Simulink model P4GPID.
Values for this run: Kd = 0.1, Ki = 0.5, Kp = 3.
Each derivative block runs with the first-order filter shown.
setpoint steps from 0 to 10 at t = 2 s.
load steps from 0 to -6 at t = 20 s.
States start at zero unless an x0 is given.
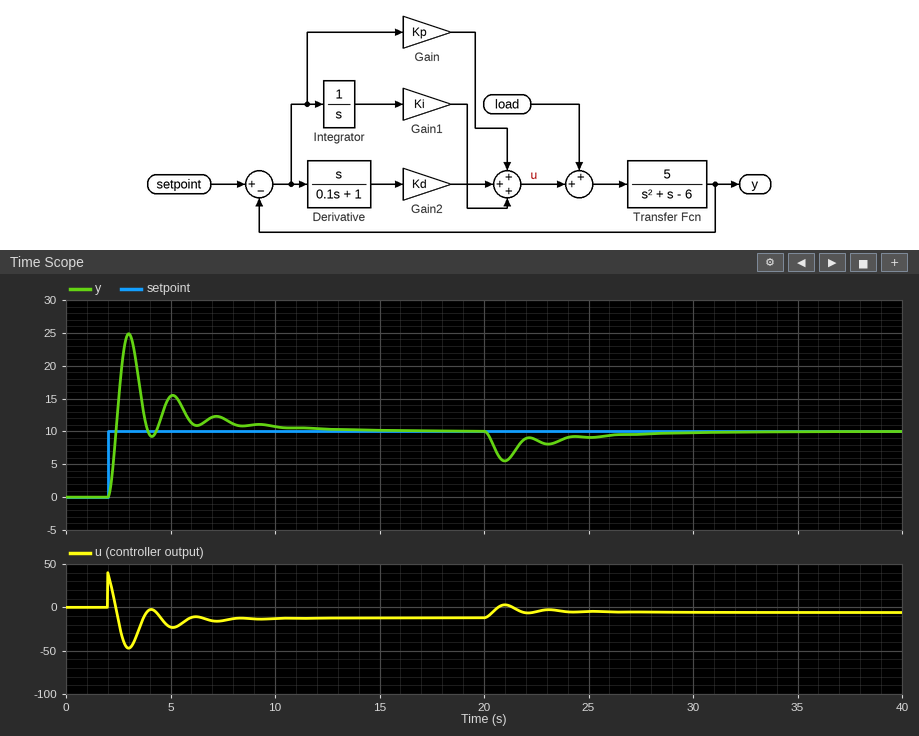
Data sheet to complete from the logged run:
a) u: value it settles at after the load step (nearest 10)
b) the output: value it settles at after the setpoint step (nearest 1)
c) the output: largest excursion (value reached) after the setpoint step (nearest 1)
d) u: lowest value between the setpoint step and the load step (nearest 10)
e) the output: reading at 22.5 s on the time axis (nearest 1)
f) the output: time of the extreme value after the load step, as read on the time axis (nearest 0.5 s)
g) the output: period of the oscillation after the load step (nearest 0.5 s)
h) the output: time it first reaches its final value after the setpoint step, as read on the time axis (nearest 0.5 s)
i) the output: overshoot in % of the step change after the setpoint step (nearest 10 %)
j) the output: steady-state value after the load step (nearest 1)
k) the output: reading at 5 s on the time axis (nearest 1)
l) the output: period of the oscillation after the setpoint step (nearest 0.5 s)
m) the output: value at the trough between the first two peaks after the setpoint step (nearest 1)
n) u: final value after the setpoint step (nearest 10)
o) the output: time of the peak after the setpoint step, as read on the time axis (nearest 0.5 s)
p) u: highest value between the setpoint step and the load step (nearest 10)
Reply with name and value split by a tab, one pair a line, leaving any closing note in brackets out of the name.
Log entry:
u: value it settles at after the load step	-10
the output: value it settles at after the setpoint step	10
the output: largest excursion (value reached) after the setpoint step	25
u: lowest value between the setpoint step and the load step	-50
the output: reading at 22.5 s on the time axis	9
the output: time of the extreme value after the load step, as read on the time axis	21.0 s
the output: period of the oscillation after the load step	2.0 s
the output: time it first reaches its final value after the setpoint step, as read on the time axis	2.5 s
the output: overshoot in % of the step change after the setpoint step	150 %
the output: steady-state value after the load step	10
the output: reading at 5 s on the time axis	15
the output: period of the oscillation after the setpoint step	2.0 s
the output: value at the trough between the first two peaks after the setpoint step	9
u: final value after the setpoint step	-10
the output: time of the peak after the setpoint step, as read on the time axis	3.0 s
u: highest value between the setpoint step and the load step	40
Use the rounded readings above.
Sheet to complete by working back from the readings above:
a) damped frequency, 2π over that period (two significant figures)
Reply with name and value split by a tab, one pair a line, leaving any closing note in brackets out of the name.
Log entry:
damped frequency, 2π over that period	3.1 rad/s
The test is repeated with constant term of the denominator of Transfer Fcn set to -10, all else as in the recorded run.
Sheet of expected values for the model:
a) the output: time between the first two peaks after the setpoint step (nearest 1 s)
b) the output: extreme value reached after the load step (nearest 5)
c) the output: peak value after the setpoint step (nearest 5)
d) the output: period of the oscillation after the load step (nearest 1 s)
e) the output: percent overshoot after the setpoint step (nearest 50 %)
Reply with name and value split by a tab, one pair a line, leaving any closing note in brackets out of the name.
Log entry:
the output: time between the first two peaks after the setpoint step	3 s
the output: extreme value reached after the load step	5
the output: peak value after the setpoint step	40
the output: period of the oscillation after the load step	3 s
the output: percent overshoot after the setpoint step	300 %
